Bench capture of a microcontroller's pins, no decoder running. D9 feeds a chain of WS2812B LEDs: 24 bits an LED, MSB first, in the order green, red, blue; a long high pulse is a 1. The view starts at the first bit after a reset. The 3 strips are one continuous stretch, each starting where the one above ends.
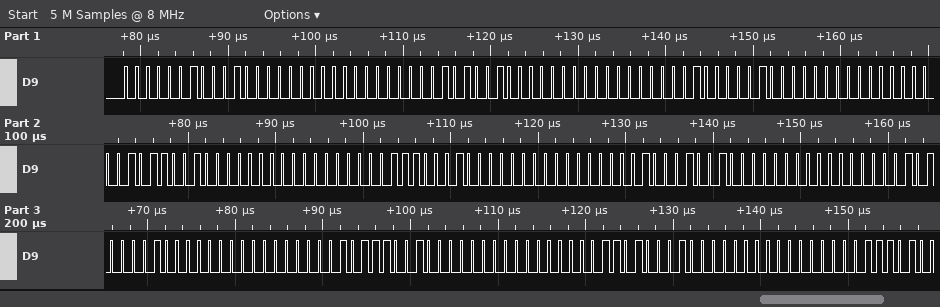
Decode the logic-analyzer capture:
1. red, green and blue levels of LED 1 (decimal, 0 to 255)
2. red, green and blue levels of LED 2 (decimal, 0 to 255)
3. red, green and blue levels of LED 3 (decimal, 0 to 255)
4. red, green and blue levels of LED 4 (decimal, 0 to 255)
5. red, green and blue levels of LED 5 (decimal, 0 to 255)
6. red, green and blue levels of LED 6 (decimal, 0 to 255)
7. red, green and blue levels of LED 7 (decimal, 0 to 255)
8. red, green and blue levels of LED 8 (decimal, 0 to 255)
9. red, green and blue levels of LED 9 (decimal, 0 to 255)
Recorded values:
32, 2, 0
32, 5, 0
32, 8, 0
32, 11, 0
32, 14, 0
32, 17, 0
32, 20, 0
32, 23, 0
32, 26, 0
